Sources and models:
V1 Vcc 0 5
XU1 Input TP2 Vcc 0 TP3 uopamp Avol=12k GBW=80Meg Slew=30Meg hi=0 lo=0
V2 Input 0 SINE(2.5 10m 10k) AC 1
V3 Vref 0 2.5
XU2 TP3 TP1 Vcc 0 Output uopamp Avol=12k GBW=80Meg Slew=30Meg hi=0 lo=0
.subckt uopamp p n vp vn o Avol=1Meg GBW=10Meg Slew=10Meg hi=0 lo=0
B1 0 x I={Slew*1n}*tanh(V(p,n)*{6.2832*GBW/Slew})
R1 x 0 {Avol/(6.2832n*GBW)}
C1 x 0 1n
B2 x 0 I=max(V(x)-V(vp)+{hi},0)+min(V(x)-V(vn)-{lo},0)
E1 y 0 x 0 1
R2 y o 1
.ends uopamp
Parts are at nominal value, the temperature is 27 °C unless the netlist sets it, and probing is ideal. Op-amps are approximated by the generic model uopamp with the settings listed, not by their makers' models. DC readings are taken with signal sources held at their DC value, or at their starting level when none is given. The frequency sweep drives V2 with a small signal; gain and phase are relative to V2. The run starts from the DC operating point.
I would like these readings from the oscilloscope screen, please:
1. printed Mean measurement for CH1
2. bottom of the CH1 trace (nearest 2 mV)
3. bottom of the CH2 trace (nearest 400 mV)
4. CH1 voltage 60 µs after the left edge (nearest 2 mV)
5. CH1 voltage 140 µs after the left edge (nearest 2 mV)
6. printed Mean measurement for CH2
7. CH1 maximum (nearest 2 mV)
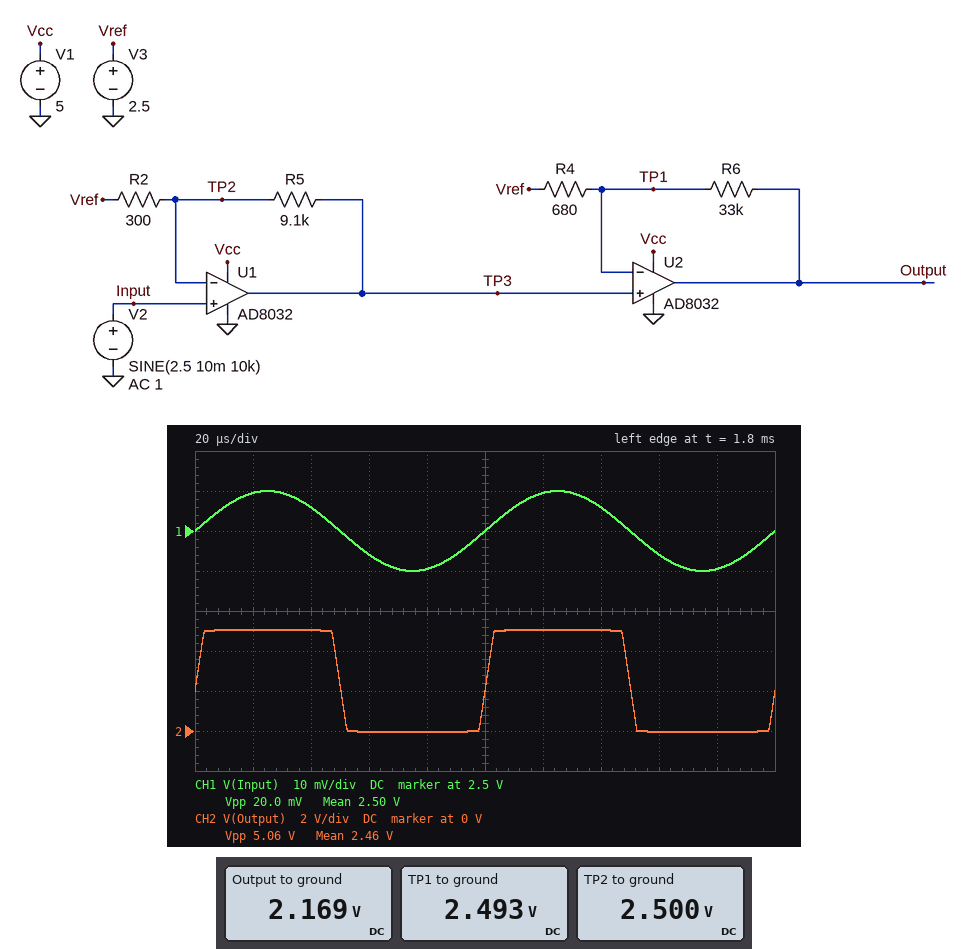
2.50 V
2.490 V
0 V
2.494 V
2.506 V
2.46 V
2.510 V
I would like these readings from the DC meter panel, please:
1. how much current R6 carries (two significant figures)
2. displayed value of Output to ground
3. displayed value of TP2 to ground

9.8 µA
2.169 V
2.500 V
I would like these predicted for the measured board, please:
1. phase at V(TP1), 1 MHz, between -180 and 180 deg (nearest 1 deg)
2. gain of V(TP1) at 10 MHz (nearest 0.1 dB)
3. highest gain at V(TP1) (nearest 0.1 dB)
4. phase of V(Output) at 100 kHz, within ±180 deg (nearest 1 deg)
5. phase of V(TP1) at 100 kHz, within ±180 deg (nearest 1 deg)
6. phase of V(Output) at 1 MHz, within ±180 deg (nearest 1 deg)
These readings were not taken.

-53 deg
1.8 dB
29.9 dB
-6 deg
-6 deg
-53 deg
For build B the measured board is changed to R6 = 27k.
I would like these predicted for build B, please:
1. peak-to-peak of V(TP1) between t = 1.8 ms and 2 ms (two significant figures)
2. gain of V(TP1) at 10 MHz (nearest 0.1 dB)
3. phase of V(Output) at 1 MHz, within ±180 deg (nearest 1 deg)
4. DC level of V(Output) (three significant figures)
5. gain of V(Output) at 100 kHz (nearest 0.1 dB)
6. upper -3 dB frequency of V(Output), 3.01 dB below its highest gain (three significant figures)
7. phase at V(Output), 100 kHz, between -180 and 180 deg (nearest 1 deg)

120 mV
3.5 dB
-48 deg
2.23 V
62.0 dB
1.43 MHz
-5 deg
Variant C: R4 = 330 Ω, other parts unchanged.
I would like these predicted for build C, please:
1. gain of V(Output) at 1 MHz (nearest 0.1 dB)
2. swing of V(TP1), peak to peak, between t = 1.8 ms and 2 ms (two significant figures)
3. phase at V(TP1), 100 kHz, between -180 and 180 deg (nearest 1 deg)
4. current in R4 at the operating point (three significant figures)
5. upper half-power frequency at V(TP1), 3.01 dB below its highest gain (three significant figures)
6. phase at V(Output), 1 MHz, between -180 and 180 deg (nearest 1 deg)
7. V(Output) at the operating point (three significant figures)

65.2 dB
50 mV
-9 deg
20.2 µA
735 kHz
-73 deg
1.83 V
